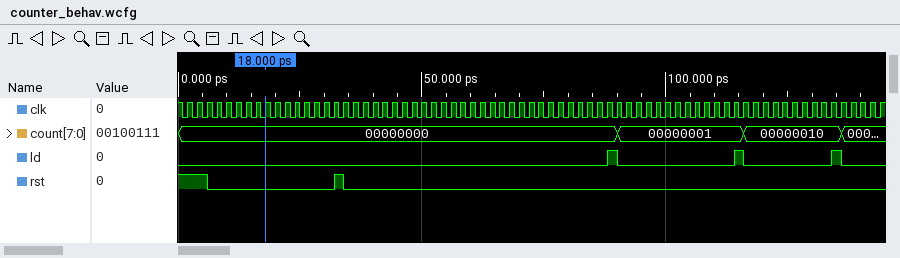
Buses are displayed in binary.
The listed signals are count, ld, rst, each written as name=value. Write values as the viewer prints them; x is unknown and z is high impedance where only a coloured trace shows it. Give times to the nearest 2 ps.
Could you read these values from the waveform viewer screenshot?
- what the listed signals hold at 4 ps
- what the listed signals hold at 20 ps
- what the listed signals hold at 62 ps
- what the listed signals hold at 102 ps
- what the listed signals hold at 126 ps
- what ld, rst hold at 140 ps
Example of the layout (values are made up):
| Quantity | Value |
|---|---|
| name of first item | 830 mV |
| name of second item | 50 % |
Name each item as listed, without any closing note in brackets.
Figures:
| Quantity | Value |
|---|---|
| what the listed signals hold at 4 ps | count=00000000, ld=0, rst=1 |
| what the listed signals hold at 20 ps | count=00000000, ld=0, rst=0 |
| what the listed signals hold at 62 ps | count=00000000, ld=0, rst=0 |
| what the listed signals hold at 102 ps | count=00000001, ld=0, rst=0 |
| what the listed signals hold at 126 ps | count=00000010, ld=0, rst=0 |
| what ld, rst hold at 140 ps | ld=0, rst=0 |
